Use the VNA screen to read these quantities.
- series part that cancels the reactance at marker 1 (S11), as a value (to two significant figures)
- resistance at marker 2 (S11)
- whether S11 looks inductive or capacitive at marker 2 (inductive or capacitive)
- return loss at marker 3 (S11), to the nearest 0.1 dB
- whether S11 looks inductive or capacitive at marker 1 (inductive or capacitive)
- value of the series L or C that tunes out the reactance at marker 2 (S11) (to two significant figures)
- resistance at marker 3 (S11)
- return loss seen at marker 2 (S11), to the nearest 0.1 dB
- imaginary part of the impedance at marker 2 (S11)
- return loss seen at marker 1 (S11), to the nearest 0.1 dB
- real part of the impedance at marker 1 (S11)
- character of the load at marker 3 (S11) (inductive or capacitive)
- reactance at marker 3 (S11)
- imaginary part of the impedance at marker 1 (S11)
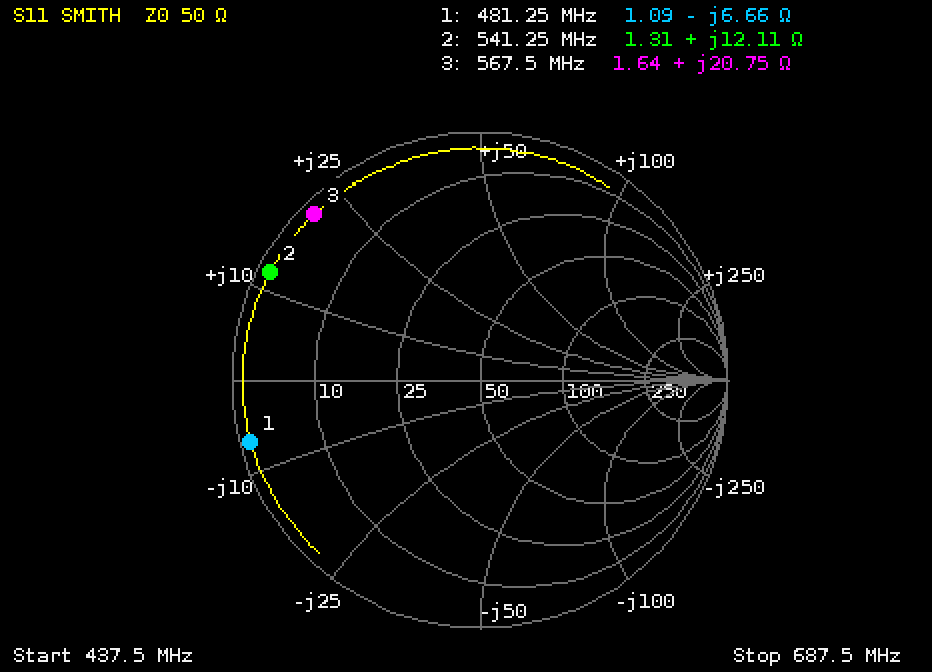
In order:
2.2 nH
1.31 Ω
inductive
0.5 dB
capacitive
24 pF
1.64 Ω
0.4 dB
+12.11 Ω
0.4 dB
1.09 Ω
inductive
+20.75 Ω
-6.66 Ω
